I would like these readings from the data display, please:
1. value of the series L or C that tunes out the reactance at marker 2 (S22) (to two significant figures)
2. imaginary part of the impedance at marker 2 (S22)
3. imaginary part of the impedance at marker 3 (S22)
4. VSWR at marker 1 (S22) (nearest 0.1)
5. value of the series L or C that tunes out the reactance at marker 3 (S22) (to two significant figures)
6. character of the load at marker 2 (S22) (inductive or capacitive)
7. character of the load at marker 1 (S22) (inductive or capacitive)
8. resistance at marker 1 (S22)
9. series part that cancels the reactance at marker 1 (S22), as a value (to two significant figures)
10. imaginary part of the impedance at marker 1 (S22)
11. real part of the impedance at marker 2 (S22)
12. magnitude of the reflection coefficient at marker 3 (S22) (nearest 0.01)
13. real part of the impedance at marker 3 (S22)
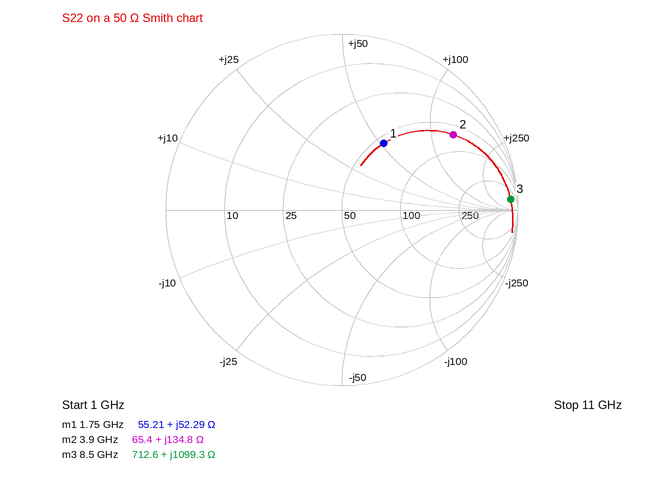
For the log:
300 fF
+134.8 Ω
+1099.3 Ω
2.6
17 fF
inductive
inductive
55.21 Ω
1.7 pF
+52.29 Ω
65.4 Ω
0.96
712.6 Ω
